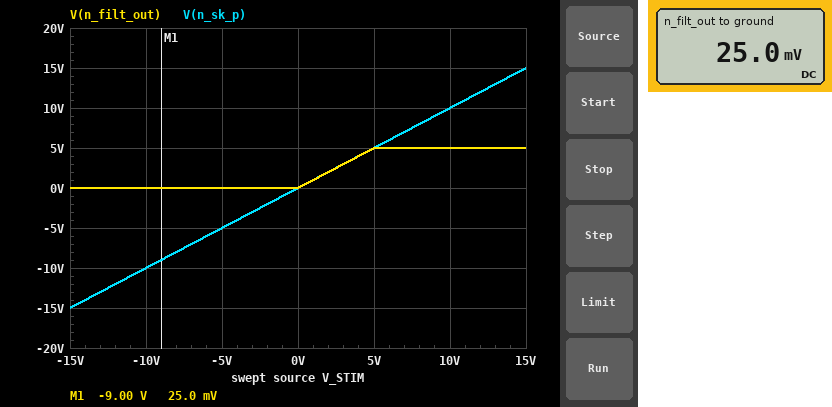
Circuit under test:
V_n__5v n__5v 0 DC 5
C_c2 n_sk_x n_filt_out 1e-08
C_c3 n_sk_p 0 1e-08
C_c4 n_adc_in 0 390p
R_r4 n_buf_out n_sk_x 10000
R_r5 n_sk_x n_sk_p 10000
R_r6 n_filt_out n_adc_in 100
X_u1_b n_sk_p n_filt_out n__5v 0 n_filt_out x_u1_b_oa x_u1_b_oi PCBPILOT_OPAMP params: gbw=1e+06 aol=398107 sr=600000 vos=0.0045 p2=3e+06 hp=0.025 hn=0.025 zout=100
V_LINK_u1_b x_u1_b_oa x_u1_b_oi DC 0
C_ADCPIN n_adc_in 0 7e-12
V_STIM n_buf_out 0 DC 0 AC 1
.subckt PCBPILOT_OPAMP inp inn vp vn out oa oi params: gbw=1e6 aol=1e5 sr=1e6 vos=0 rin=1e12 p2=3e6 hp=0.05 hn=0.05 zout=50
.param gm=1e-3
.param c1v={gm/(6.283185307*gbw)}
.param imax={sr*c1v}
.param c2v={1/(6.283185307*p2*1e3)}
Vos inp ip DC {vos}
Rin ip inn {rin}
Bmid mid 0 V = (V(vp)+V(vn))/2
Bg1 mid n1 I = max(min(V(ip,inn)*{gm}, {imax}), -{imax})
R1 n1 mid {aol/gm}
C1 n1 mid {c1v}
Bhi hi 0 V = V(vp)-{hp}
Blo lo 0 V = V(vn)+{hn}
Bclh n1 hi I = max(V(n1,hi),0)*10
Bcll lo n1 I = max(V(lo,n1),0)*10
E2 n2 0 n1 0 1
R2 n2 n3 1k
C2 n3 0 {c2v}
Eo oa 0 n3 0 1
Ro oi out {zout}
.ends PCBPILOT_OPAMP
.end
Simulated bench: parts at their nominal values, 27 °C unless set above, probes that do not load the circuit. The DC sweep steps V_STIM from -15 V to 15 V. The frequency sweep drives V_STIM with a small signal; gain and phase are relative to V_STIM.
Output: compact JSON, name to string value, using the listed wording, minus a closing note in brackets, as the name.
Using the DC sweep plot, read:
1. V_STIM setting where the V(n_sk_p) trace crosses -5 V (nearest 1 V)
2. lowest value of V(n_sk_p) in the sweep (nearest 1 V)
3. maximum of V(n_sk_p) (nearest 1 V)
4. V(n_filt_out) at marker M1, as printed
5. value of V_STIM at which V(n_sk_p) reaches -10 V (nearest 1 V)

{"V_STIM setting where the V(n_sk_p) trace crosses -5 V": "-5 V", "lowest value of V(n_sk_p) in the sweep": "-15 V", "maximum of V(n_sk_p)": "15 V", "V(n_filt_out) at marker M1, as printed": "25.0 mV", "value of V_STIM at which V(n_sk_p) reaches -10 V": "-10 V"}
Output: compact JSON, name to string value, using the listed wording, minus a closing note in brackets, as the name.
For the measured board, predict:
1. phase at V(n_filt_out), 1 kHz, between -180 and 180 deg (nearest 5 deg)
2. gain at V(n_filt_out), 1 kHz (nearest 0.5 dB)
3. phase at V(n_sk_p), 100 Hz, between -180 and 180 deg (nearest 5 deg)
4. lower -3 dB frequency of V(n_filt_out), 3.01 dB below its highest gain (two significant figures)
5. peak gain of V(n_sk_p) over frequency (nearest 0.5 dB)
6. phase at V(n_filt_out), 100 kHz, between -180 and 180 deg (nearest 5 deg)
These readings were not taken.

{"phase at V(n_filt_out), 1 kHz, between -180 and 180 deg": "50 deg", "gain at V(n_filt_out), 1 kHz": "-48.5 dB", "phase at V(n_sk_p), 100 Hz, between -180 and 180 deg": "-10 deg", "lower -3 dB frequency of V(n_filt_out), 3.01 dB below its highest gain": "3.5 kHz", "peak gain of V(n_sk_p) over frequency": "0 dB", "phase at V(n_filt_out), 100 kHz, between -180 and 180 deg": "0 deg"}
